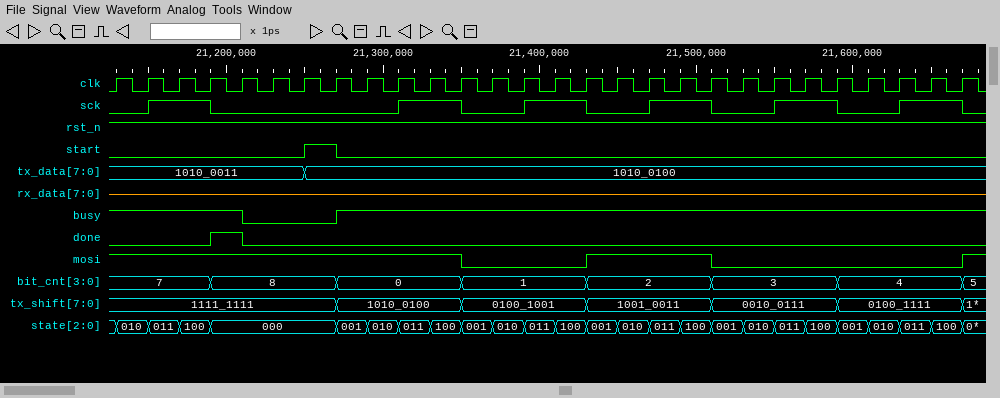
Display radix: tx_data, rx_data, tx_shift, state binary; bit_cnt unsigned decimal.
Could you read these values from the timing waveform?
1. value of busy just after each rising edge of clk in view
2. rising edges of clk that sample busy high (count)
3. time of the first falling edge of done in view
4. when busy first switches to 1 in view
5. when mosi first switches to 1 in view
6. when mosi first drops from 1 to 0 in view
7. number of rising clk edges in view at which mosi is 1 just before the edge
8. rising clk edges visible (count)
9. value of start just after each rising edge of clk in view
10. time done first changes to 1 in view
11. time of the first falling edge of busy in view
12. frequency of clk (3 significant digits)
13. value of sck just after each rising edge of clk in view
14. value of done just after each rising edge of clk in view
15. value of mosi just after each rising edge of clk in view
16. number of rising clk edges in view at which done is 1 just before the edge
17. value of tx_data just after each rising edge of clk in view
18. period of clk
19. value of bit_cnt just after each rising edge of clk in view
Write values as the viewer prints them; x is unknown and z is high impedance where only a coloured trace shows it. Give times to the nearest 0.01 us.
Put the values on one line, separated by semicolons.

1 1 1 1 0 0 0 1 1 1 1 1 1 1 1 1 1 1 1 1 1 1 1 1 1 1 1 1; 25; 21.21 us; 21.27 us; 21.43 us; 21.35 us; 16; 28; 0 0 0 0 0 0 1 0 0 0 0 0 0 0 0 0 0 0 0 0 0 0 0 0 0 0 0 0; 21.19 us; 21.21 us; 50.0 MHz; 0 1 1 0 0 0 0 0 0 1 1 0 0 1 1 0 0 1 1 0 0 1 1 0 0 1 1 0; 0 0 0 1 0 0 0 0 0 0 0 0 0 0 0 0 0 0 0 0 0 0 0 0 0 0 0 0; 1 1 1 1 1 1 1 1 1 1 1 0 0 0 0 1 1 1 1 0 0 0 0 0 0 0 0 1; 1; 1010_0011, 1010_0011, 1010_0011, 1010_0011, 1010_0011, 1010_0011, 1010_0100, 1010_0100, 1010_0100, 1010_0100, 1010_0100, 1010_0100, 1010_0100, 1010_0100, 1010_0100, 1010_0100, 1010_0100, 1010_0100, 1010_0100, 1010_0100, 1010_0100, 1010_0100, 1010_0100, 1010_0100, 1010_0100, 1010_0100, 1010_0100, 1010_0100; 0.02 us; 7, 7, 7, 8, 8, 8, 8, 0, 0, 0, 0, 1, 1, 1, 1, 2, 2, 2, 2, 3, 3, 3, 3, 4, 4, 4, 4, 5
